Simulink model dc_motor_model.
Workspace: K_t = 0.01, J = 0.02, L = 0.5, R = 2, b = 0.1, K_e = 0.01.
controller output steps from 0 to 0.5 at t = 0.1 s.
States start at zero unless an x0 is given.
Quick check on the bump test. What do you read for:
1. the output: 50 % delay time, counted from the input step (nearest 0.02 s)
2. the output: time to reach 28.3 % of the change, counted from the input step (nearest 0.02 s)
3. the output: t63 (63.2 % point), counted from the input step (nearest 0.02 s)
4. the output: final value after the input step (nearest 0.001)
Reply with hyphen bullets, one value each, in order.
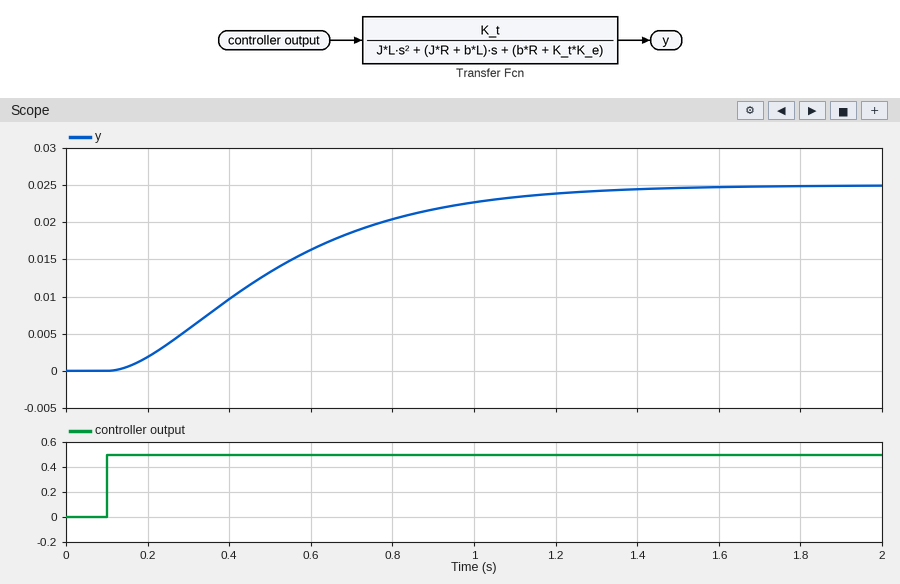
- 0.38 s
- 0.24 s
- 0.48 s
- 0.025
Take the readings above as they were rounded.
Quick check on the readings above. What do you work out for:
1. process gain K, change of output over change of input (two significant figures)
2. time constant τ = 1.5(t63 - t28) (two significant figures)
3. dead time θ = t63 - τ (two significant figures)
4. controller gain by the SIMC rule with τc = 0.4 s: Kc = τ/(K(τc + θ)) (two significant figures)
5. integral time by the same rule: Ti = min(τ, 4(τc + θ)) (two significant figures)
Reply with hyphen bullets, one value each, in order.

- 0.050
- 0.36 s
- 0.12 s
- 14
- 0.36 s
